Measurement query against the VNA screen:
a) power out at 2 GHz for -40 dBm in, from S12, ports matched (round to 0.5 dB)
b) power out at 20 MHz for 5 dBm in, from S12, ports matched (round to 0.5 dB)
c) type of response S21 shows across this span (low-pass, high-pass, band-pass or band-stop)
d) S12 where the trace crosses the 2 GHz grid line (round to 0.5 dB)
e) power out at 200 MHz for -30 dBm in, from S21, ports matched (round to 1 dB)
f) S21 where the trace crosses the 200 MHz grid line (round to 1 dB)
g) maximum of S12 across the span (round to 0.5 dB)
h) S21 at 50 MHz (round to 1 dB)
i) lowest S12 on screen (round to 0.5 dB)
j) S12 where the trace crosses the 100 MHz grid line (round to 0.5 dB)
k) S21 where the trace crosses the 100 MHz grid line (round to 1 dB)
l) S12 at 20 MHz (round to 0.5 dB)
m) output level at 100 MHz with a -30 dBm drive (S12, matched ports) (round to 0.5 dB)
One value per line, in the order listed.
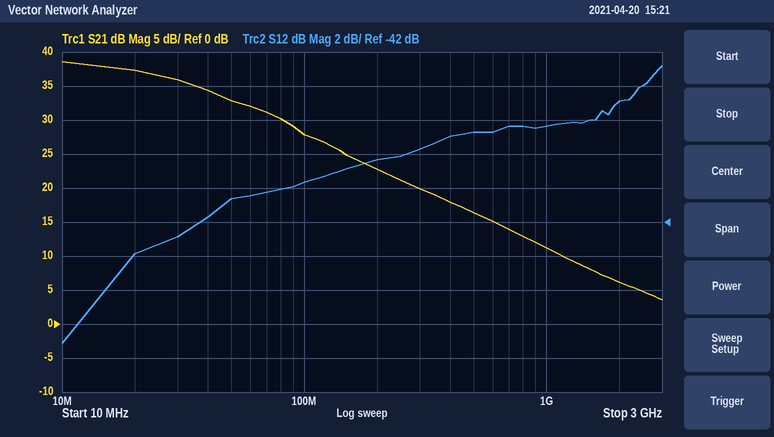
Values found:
-75.0 dBm
-39.0 dBm
low-pass
-35.0 dB
-7 dBm
23 dB
-33.0 dB
33 dB
-49.0 dB
-39.5 dB
28 dB
-44.0 dB
-69.5 dBm
